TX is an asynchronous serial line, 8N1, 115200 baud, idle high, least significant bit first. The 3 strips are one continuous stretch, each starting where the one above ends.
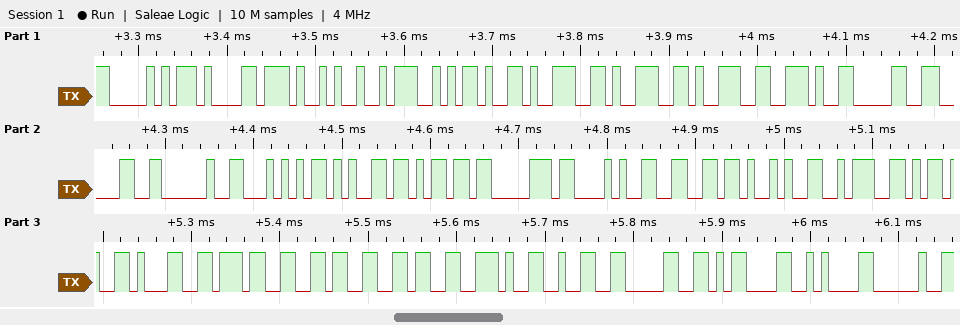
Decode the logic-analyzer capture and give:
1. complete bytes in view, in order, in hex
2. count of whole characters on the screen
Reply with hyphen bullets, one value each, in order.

- 50 61 29 3A 2D 39 39 39 2E 30 30 20 54 65 6D 70 28 66 29 3A 2D 31 37 36 36 2E 32 30 0D 0A 20
- 31
